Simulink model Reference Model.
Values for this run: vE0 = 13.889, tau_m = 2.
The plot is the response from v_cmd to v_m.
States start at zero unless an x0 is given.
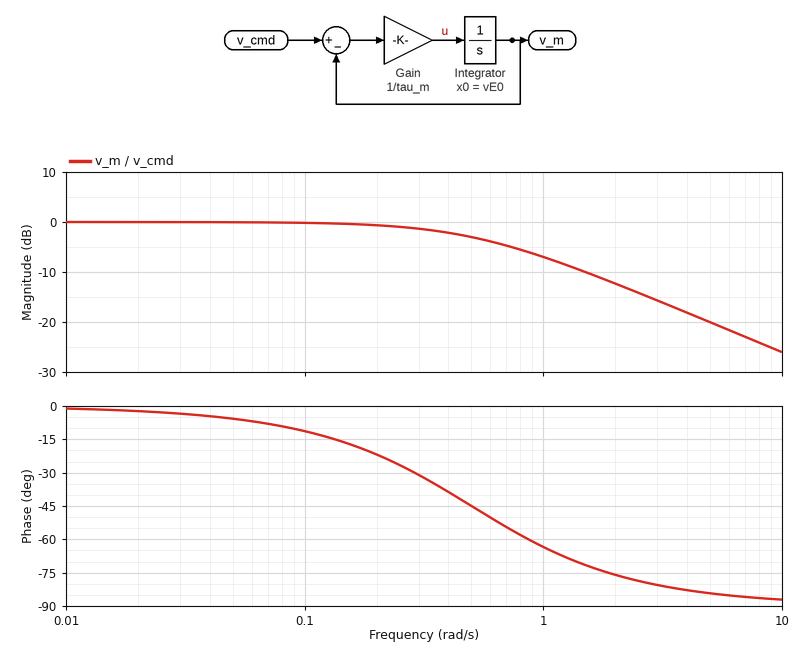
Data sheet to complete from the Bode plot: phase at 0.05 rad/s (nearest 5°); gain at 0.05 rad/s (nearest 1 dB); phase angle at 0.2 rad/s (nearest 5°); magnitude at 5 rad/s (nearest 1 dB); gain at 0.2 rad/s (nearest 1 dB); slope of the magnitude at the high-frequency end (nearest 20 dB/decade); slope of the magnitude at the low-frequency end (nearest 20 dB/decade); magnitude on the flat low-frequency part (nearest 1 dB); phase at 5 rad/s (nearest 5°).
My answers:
-5°
0 dB
-20°
-20 dB
-1 dB
-20 dB/decade
0 dB/decade
0 dB
-85°
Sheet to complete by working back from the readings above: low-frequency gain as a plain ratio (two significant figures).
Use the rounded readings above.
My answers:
1.0
